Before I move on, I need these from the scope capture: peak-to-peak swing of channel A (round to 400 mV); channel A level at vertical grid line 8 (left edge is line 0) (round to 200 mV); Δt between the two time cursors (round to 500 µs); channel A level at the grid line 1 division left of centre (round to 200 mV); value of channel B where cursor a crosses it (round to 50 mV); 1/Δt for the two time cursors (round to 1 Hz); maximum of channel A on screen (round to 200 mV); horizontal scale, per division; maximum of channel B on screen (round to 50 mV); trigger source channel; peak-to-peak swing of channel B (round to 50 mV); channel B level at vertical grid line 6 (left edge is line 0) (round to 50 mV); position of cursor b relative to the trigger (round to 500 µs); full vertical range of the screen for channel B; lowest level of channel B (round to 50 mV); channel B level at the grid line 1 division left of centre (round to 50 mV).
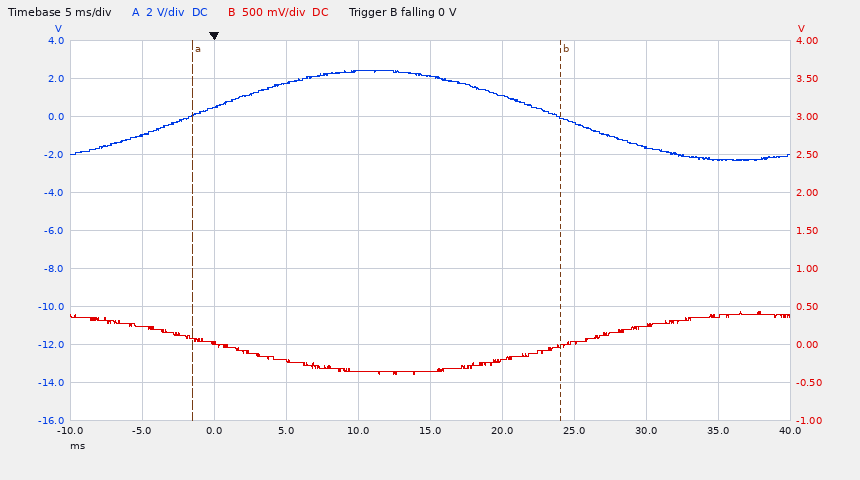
4.8 V
-1.6 V
25.5 ms
2.4 V
100 mV
39 Hz
2.4 V
5 ms
450 mV
channel B
850 mV
-200 mV
+24.0 ms
5 V
-400 mV
-350 mV
